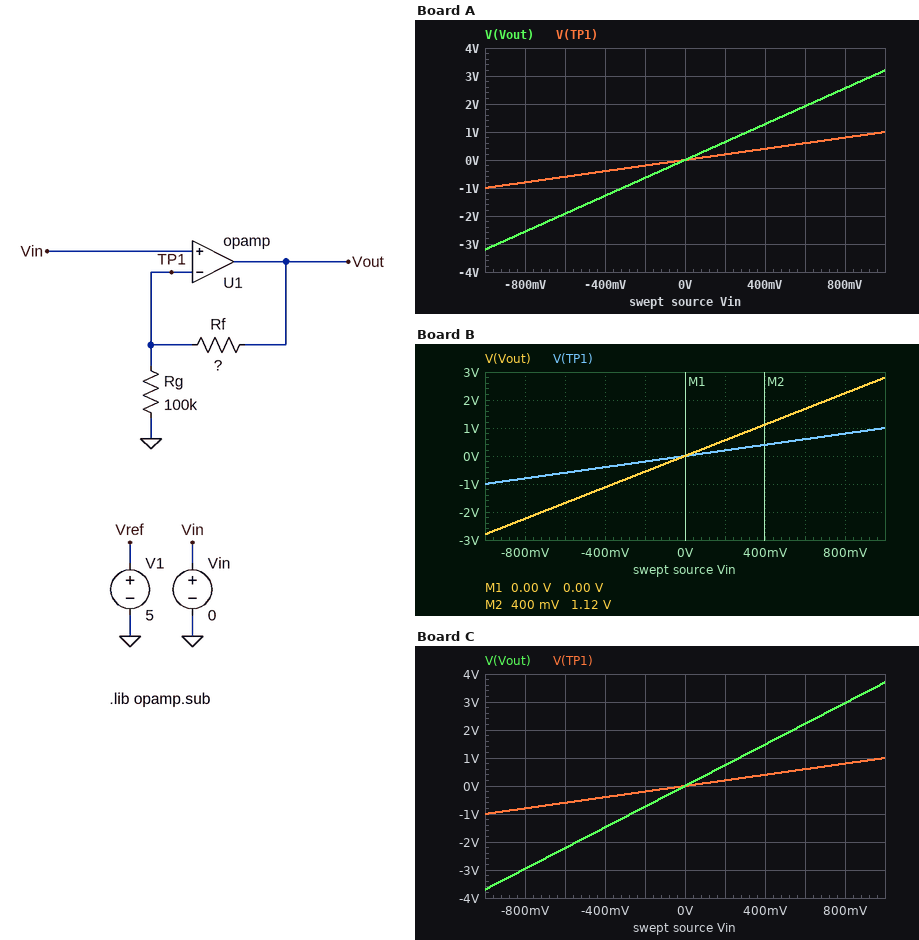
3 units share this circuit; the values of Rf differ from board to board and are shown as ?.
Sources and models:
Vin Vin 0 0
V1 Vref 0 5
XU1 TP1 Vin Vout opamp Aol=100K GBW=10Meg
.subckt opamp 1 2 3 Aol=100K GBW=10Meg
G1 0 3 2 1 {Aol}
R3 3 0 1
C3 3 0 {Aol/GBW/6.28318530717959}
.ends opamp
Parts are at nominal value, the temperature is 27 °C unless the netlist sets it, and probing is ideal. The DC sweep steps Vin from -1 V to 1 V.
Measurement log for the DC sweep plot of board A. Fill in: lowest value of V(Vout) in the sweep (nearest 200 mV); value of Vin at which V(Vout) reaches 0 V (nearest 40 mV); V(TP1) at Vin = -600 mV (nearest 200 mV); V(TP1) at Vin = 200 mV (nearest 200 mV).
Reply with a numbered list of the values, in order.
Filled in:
1. -3.2 V
2. 0 V
3. -600 mV
4. 200 mV
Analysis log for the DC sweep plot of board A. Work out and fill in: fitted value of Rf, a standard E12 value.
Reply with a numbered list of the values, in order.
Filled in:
1. 220 kΩ
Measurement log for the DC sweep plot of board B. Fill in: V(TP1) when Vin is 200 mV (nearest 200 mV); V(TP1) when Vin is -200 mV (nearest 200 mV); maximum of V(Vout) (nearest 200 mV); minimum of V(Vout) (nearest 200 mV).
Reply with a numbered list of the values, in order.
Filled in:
1. 200 mV
2. -200 mV
3. 2.8 V
4. -2.8 V
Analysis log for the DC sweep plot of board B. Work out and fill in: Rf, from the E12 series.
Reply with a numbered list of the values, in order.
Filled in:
1. 180 kΩ
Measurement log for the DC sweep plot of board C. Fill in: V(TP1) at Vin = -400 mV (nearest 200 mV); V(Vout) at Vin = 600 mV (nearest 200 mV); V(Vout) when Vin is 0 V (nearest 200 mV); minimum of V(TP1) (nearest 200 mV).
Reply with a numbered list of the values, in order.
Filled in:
1. -400 mV
2. 2.2 V
3. 0 V
4. -1.0 V
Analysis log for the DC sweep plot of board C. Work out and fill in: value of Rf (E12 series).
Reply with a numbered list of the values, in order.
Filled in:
1. 270 kΩ
